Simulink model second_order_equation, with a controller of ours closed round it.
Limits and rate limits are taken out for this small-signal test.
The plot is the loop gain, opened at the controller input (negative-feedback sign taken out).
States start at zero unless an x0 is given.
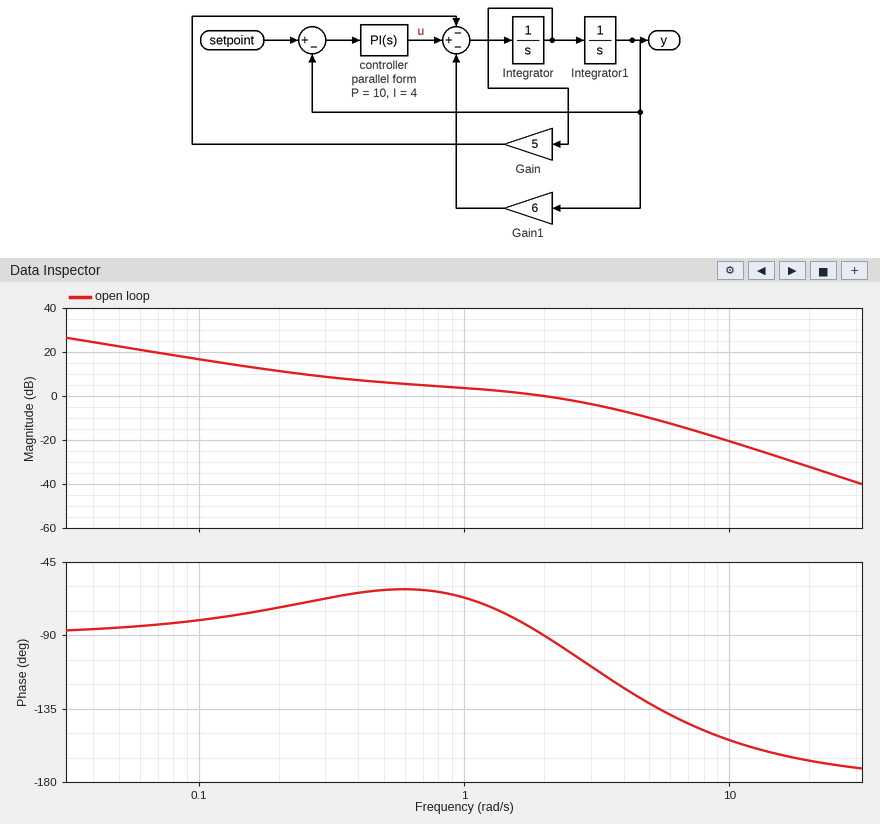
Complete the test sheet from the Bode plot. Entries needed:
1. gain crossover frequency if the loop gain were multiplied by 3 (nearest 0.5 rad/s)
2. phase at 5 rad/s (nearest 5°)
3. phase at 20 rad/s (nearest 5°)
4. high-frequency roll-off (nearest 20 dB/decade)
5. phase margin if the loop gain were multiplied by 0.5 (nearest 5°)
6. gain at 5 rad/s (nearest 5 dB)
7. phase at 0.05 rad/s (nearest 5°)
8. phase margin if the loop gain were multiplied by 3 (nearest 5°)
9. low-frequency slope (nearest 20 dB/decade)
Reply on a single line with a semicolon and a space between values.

5.0 rad/s; -130°; -165°; -40 dB/decade; 120°; -10 dB; -85°; 50°; -20 dB/decade
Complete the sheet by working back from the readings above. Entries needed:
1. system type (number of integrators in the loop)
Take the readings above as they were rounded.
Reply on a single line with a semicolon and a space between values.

1
